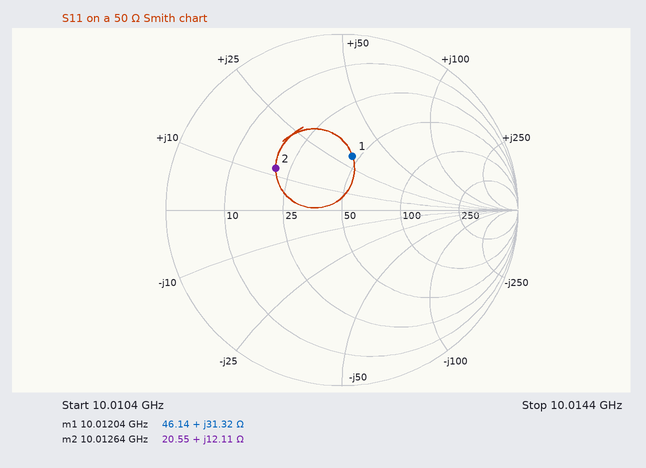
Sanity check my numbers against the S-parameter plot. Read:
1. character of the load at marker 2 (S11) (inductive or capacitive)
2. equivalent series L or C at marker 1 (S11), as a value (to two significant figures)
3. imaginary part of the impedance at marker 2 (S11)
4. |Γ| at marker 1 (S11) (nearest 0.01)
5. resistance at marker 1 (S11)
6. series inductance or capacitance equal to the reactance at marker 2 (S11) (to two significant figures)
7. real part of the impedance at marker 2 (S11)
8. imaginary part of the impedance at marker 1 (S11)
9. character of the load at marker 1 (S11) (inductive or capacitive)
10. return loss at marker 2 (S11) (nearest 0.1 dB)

inductive
500 pH
+12.11 Ω
0.31
46.14 Ω
190 pH
20.55 Ω
+31.32 Ω
inductive
7.0 dB
